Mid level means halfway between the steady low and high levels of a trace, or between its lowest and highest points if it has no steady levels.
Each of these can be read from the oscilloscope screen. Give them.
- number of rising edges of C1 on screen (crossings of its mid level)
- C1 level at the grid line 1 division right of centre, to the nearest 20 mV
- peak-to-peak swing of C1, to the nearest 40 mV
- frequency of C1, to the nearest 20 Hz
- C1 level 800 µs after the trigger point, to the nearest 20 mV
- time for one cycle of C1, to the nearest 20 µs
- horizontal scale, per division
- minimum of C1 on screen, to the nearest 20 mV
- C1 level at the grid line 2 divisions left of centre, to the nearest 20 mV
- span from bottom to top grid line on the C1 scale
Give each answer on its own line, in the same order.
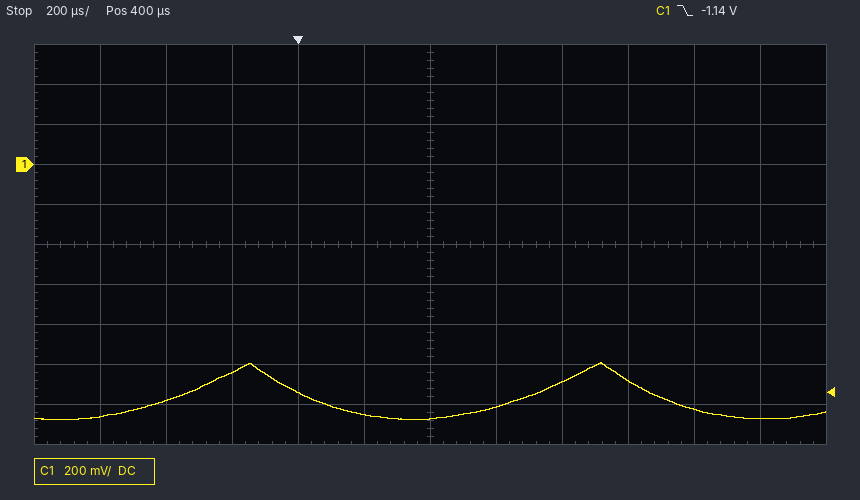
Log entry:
2
-1.22 V
280 mV
940 Hz
-1.08 V
1.06 ms
200 µs
-1.28 V
-1.14 V
2 V
